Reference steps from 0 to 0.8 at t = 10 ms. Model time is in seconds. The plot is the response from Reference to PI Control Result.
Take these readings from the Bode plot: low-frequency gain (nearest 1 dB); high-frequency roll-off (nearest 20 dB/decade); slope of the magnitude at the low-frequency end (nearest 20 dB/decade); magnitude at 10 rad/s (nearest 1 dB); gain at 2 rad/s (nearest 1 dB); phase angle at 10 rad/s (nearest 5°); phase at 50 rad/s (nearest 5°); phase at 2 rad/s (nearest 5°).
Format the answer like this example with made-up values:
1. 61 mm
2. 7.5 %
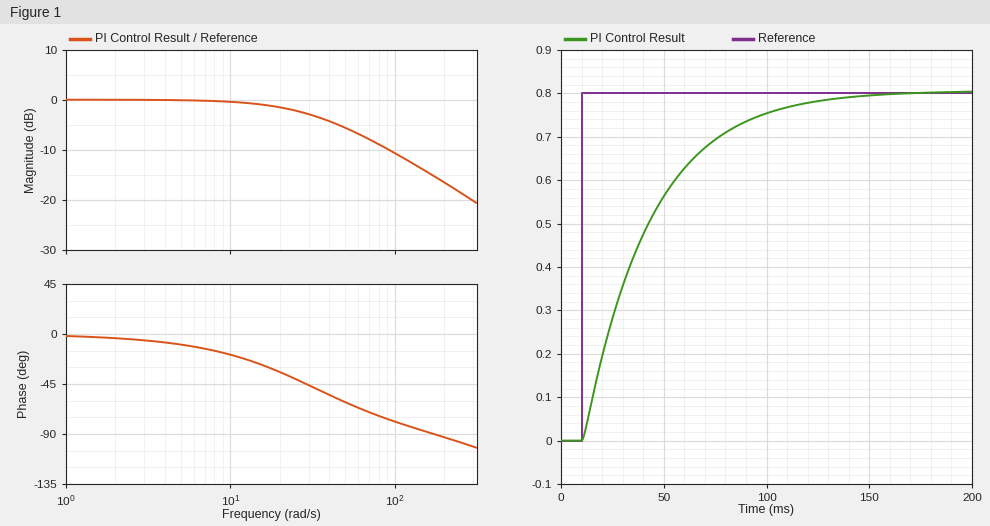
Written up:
1. 0 dB
2. -20 dB/decade
3. 0 dB/decade
4. 0 dB
5. 0 dB
6. -20°
7. -60°
8. -5°
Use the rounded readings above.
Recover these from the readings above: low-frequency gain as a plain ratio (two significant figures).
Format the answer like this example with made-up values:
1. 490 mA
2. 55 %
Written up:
1. 1.0
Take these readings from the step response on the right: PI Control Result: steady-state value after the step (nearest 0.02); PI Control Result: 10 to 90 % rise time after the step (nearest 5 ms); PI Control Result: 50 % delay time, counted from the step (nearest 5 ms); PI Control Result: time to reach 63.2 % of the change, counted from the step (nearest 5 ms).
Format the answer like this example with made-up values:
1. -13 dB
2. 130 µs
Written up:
1. 0.80
2. 70 ms
3. 25 ms
4. 35 ms
